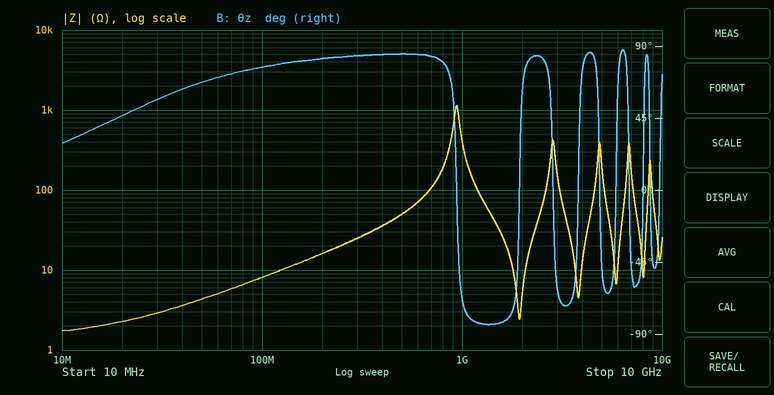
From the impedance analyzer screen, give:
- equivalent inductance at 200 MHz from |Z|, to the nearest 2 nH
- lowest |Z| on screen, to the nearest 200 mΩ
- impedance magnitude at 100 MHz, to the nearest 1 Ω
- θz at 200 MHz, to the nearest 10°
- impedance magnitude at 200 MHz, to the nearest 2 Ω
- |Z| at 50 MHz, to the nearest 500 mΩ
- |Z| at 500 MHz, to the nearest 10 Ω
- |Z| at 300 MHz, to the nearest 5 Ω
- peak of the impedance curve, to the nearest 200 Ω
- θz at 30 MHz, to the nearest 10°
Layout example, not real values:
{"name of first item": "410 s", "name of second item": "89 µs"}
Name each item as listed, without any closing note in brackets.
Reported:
{"equivalent inductance at 200 MHz from |Z|, to the nearest 2 nH": "12 nH", "lowest |Z| on screen, to the nearest 200 mΩ": "1.8 Ω", "impedance magnitude at 100 MHz, to the nearest 1 Ω": "8 Ω", "θz at 200 MHz, to the nearest 10°": "80°", "impedance magnitude at 200 MHz, to the nearest 2 Ω": "16 Ω", "|Z| at 50 MHz, to the nearest 500 mΩ": "4.5 Ω", "|Z| at 500 MHz, to the nearest 10 Ω": "50 Ω", "|Z| at 300 MHz, to the nearest 5 Ω": "25 Ω", "peak of the impedance curve, to the nearest 200 Ω": "1.2 kΩ", "θz at 30 MHz, to the nearest 10°": "60°"}
